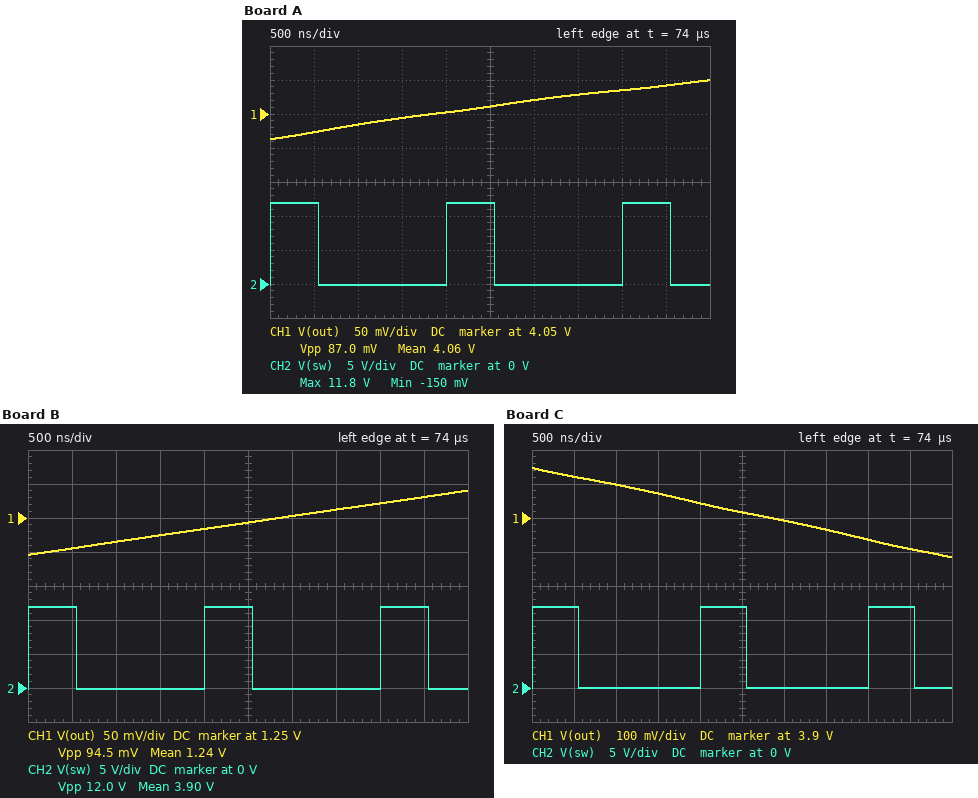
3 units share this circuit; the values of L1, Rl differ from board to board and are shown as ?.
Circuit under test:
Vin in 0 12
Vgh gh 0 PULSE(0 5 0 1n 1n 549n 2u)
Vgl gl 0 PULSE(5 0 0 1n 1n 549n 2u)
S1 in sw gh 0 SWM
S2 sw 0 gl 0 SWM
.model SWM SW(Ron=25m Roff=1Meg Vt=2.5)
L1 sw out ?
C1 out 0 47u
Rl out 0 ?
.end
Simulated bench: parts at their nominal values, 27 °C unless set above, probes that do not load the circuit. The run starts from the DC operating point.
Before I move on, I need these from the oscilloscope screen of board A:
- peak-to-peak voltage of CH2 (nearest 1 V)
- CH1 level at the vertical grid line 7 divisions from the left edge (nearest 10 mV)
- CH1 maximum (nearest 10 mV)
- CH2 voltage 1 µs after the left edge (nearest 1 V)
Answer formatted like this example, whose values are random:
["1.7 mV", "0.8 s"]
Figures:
["12 V", "4.08 V", "4.10 V", "0 V"]
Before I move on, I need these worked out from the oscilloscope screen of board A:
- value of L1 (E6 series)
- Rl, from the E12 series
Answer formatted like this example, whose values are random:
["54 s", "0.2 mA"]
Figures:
["15 µH", "0.82 Ω"]
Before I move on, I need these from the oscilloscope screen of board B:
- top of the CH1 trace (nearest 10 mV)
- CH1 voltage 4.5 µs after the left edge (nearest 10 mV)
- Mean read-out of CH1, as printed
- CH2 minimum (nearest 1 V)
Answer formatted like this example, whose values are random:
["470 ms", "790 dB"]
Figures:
["1.29 V", "1.28 V", "1.24 V", "0 V"]
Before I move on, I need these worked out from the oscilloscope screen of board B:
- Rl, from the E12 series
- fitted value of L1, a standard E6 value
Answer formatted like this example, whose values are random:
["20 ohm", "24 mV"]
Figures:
["0.56 Ω", "68 µH"]
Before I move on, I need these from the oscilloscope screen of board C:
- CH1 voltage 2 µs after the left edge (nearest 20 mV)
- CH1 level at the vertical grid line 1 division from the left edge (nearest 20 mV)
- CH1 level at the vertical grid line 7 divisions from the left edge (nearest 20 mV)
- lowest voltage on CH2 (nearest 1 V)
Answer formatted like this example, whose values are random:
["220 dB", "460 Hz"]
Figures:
["3.94 V", "4.02 V", "3.86 V", "0 V"]
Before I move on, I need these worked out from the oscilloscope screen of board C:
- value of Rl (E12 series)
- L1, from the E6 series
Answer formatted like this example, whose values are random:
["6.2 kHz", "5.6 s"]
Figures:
["0.82 Ω", "6.8 µH"]
